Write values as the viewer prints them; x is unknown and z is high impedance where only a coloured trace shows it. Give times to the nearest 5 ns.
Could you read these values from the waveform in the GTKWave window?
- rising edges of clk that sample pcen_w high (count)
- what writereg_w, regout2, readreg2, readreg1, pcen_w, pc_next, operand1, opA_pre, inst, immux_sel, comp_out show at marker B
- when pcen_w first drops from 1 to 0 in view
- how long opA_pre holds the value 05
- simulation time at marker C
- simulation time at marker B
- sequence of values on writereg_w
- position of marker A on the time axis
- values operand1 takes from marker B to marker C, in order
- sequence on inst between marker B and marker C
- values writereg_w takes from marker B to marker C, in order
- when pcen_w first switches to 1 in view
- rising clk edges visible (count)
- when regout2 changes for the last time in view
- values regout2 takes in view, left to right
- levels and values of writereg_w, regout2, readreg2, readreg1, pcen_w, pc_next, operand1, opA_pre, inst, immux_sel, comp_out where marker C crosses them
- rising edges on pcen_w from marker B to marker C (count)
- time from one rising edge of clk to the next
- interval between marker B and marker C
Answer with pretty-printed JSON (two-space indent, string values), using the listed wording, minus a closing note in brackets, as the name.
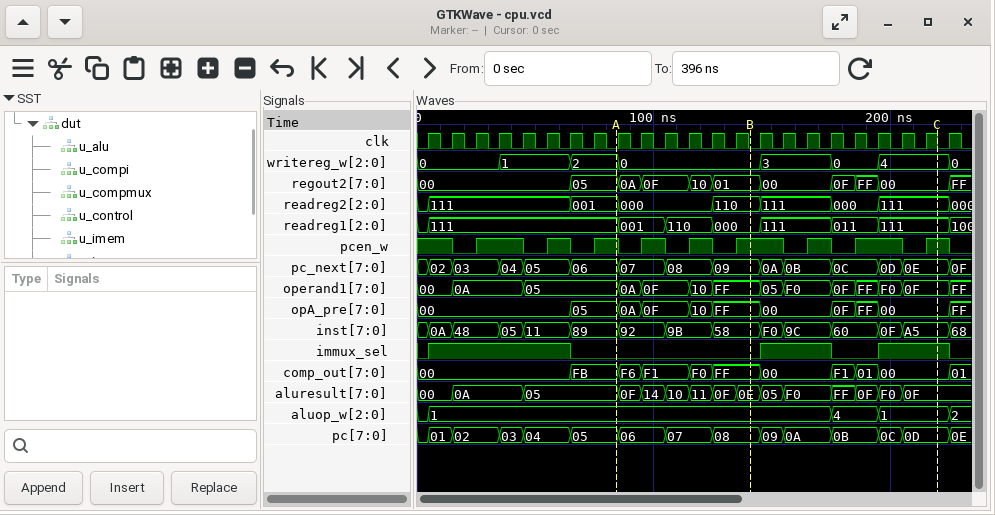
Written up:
{
  "rising edges of clk that sample pcen_w high": "14",
  "what writereg_w, regout2, readreg2, readreg1, pcen_w, pc_next, operand1, opA_pre, inst, immux_sel, comp_out show at marker B": "writereg_w=0, regout2=01, readreg2=110, readreg1=000, pcen_w=1, pc_next=09, operand1=FF, opA_pre=FF, inst=58, immux_sel=0, comp_out=FF",
  "when pcen_w first drops from 1 to 0 in view": "15 ns",
  "how long opA_pre holds the value 05": "20 ns",
  "simulation time at marker C": "220 ns",
  "simulation time at marker B": "140 ns",
  "sequence of values on writereg_w": "0, 1, 2, 0, 3, 0, 4, 0",
  "position of marker A on the time axis": "85 ns",
  "values operand1 takes from marker B to marker C, in order": "FF, 05, F0, 0F, FF, F0, 0F",
  "sequence on inst between marker B and marker C": "58, F0, 9C, 60, 0F, A5",
  "values writereg_w takes from marker B to marker C, in order": "0, 3, 0, 4",
  "when pcen_w first switches to 1 in view": "25 ns",
  "rising clk edges visible": "23",
  "when regout2 changes for the last time in view": "225 ns",
  "values regout2 takes in view, left to right": "00, 05, 0A, 0F, 10, 01, 00, 0F, FF, 00, FF",
  "levels and values of writereg_w, regout2, readreg2, readreg1, pcen_w, pc_next, operand1, opA_pre, inst, immux_sel, comp_out where marker C crosses them": "writereg_w=4, regout2=00, readreg2=111, readreg1=111, pcen_w=1, pc_next=0E, operand1=0F, opA_pre=00, inst=A5, immux_sel=1, comp_out=00",
  "rising edges on pcen_w from marker B to marker C": "3",
  "time from one rising edge of clk to the next": "10 ns",
  "interval between marker B and marker C": "80 ns"
}
